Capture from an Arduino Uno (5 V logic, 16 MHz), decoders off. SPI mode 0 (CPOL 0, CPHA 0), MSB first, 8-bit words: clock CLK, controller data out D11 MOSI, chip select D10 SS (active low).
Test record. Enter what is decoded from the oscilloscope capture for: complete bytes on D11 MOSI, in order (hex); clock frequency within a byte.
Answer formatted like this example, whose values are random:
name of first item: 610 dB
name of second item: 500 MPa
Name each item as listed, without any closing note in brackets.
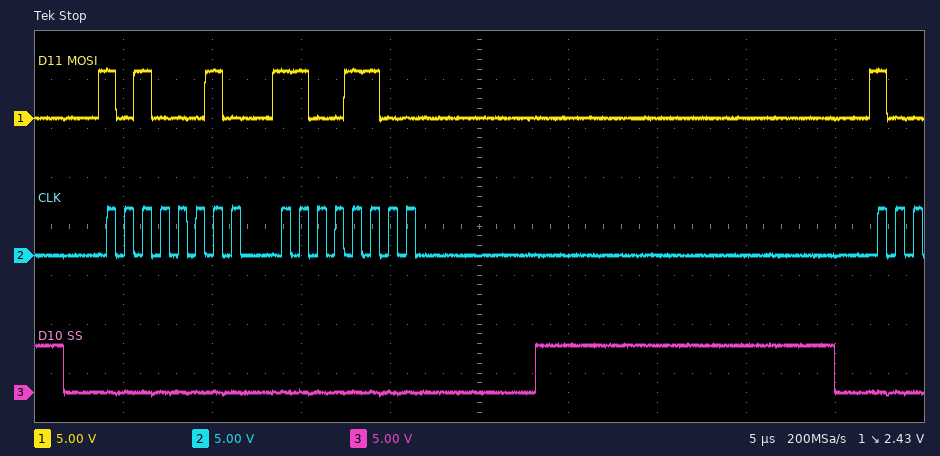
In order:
complete bytes on D11 MOSI, in order: A2 CC
clock frequency within a byte: 1 MHz
